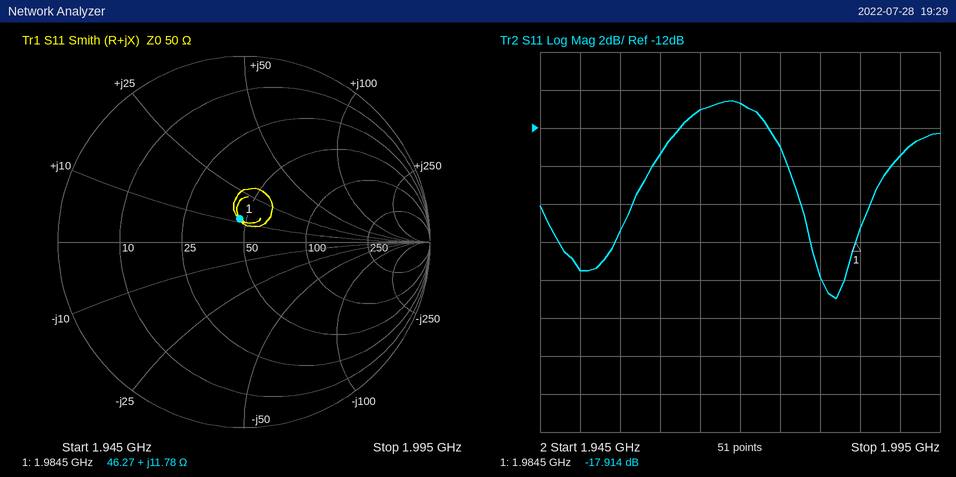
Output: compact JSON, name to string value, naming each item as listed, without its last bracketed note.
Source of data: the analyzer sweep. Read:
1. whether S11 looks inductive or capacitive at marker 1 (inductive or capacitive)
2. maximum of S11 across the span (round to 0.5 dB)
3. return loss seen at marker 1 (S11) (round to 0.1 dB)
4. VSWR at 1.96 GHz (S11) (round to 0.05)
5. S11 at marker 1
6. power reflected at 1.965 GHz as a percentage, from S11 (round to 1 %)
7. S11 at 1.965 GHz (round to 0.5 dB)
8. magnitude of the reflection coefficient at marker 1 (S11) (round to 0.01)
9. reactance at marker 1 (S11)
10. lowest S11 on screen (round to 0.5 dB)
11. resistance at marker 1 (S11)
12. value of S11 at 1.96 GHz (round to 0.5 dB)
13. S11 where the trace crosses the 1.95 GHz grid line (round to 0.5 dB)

{"whether S11 looks inductive or capacitive at marker 1": "inductive", "maximum of S11 across the span": "-10.5 dB", "return loss seen at marker 1 (S11)": "17.9 dB", "VSWR at 1.96 GHz (S11)": "1.55", "S11 at marker 1": "-17.914 dB", "power reflected at 1.965 GHz as a percentage, from S11": "8 %", "S11 at 1.965 GHz": "-11.0 dB", "magnitude of the reflection coefficient at marker 1 (S11)": "0.13", "reactance at marker 1": "+11.78 Ω", "lowest S11 on screen": "-21.0 dB", "resistance at marker 1": "46.27 Ω", "value of S11 at 1.96 GHz": "-13.5 dB", "S11 where the trace crosses the 1.95 GHz grid line": "-19.5 dB"}
